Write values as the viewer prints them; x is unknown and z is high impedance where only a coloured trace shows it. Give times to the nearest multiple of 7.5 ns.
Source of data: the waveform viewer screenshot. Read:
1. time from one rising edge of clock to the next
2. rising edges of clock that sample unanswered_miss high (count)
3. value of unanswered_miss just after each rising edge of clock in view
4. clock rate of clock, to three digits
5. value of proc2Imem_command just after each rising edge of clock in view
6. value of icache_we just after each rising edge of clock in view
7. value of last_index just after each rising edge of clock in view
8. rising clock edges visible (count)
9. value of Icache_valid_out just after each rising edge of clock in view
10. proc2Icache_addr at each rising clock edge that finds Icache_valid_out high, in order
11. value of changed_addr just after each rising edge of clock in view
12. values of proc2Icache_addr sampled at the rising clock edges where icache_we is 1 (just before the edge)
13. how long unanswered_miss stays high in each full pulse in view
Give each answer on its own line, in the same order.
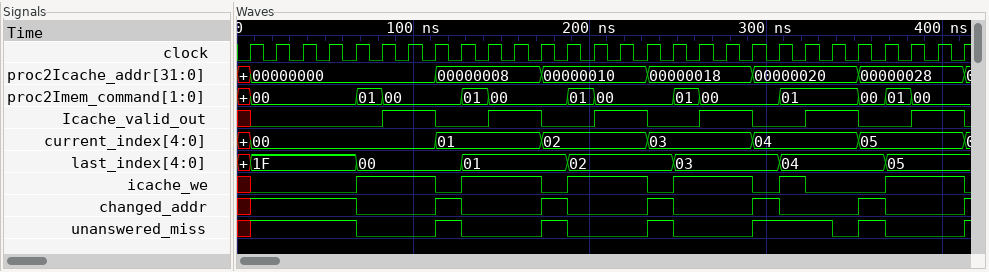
15 ns
11
1 1 1 1 0 0 0 1 0 0 0 1 0 0 0 1 0 0 0 1 1 1 0 1 0 0 0 1
66.7 MHz
00, 00, 00, 00, 01, 00, 00, 00, 01, 00, 00, 00, 01, 00, 00, 00, 01, 00, 00, 00, 01, 01, 01, 00, 01, 00, 00, 00
0 0 0 0 1 1 1 0 1 1 1 0 1 1 1 0 1 1 1 0 1 0 0 0 1 1 1 0
1F, 1F, 1F, 1F, 00, 00, 00, 00, 01, 01, 01, 01, 02, 02, 02, 02, 03, 03, 03, 03, 04, 04, 04, 04, 05, 05, 05, 05
28
0 0 0 0 0 1 1 0 0 1 1 0 0 1 1 0 0 1 1 0 0 1 1 0 0 1 1 0
00000000, 00000000, 00000008, 00000008, 00000010, 00000010, 00000018, 00000018, 00000020, 00000020, 00000028, 00000028
1 1 1 1 0 0 0 1 0 0 0 1 0 0 0 1 0 0 0 1 0 0 0 1 0 0 0 1
00000000, 00000000, 00000000, 00000008, 00000008, 00000008, 00000010, 00000010, 00000010, 00000018, 00000018, 00000018, 00000020, 00000028, 00000028, 00000028
15 ns, 15 ns, 15 ns, 45 ns, 15 ns
